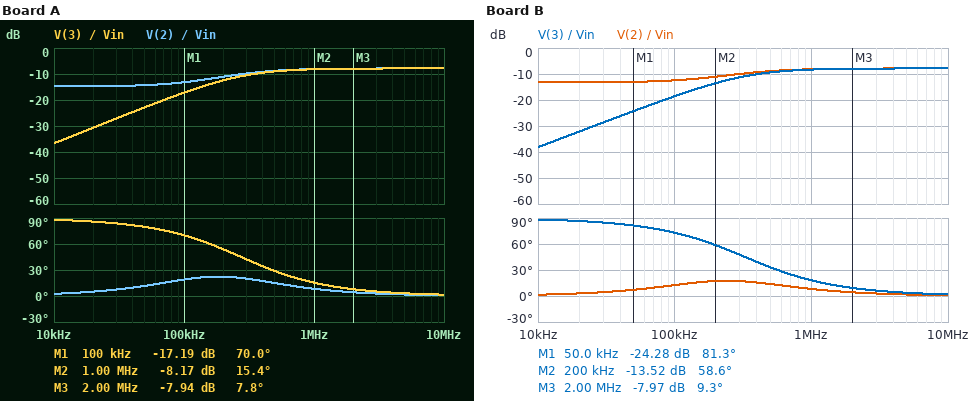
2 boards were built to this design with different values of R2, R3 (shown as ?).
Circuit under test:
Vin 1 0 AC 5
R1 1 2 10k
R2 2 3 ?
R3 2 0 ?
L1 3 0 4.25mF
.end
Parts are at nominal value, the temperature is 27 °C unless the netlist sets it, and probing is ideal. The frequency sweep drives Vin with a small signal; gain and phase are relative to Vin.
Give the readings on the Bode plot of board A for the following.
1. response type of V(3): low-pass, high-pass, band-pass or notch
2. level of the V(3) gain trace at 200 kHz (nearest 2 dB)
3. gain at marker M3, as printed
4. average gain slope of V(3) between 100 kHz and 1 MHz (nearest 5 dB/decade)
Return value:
high-pass
-12 dB
-7.94 dB
10 dB/decade
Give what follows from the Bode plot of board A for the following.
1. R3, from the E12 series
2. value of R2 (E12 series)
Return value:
6.8 kΩ
3.3 kΩ
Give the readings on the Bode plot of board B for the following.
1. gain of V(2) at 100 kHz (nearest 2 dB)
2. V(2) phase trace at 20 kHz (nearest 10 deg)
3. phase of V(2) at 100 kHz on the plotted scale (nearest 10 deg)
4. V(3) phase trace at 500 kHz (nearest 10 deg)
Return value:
-12 dB
0 deg
10 deg
30 deg
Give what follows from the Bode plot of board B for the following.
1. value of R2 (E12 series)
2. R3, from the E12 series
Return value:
4.7 kΩ
6.8 kΩ
